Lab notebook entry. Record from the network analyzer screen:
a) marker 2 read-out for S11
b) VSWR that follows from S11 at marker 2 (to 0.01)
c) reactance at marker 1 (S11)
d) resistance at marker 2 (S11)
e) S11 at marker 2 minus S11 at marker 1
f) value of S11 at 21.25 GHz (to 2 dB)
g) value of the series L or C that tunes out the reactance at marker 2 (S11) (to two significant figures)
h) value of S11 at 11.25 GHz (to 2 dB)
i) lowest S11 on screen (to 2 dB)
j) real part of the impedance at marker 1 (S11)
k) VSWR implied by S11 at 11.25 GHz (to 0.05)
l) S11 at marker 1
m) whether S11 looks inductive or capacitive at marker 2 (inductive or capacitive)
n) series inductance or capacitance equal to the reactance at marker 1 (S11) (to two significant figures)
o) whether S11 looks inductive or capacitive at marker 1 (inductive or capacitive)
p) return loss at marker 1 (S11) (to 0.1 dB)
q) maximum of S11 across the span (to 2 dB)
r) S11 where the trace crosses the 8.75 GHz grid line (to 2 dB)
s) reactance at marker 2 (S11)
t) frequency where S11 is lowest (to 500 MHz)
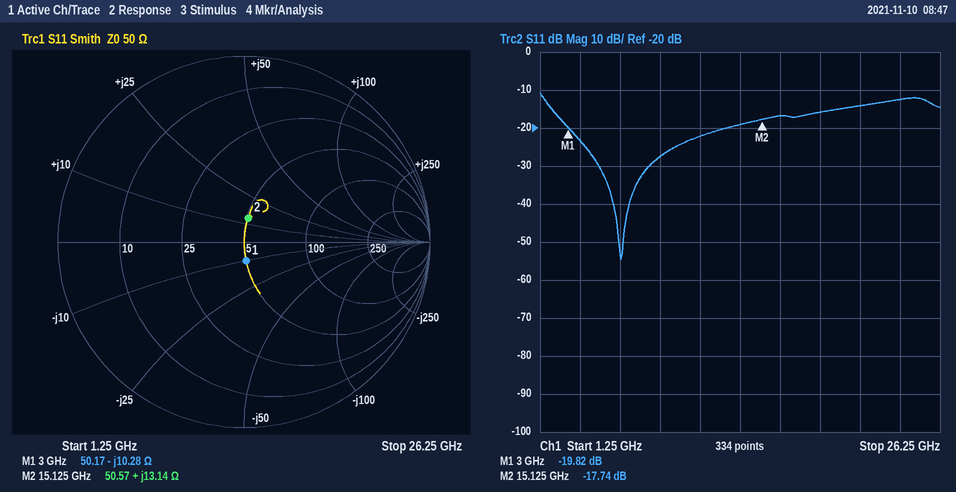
-17.74 dB
1.30
-10.28 Ω
50.57 Ω
2.08 dB
-14 dB
800 fF
-22 dB
-54 dB
50.17 Ω
1.15
-19.82 dB
inductive
5.2 pF
capacitive
19.8 dB
-10 dB
-28 dB
+13.14 Ω
6.5 GHz
